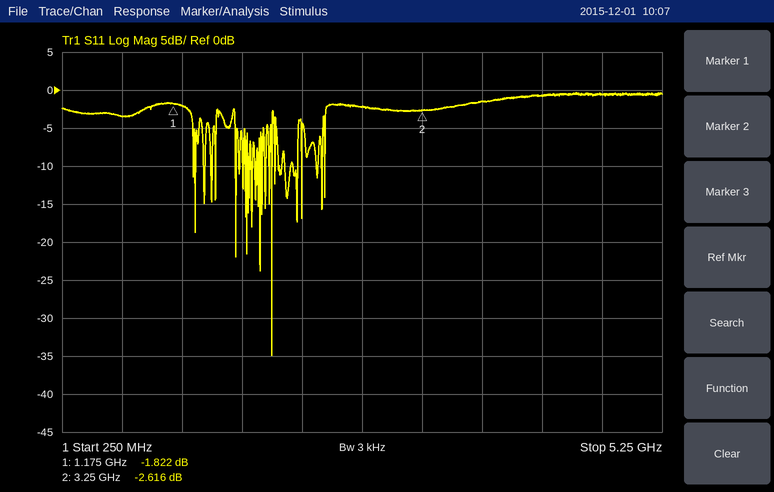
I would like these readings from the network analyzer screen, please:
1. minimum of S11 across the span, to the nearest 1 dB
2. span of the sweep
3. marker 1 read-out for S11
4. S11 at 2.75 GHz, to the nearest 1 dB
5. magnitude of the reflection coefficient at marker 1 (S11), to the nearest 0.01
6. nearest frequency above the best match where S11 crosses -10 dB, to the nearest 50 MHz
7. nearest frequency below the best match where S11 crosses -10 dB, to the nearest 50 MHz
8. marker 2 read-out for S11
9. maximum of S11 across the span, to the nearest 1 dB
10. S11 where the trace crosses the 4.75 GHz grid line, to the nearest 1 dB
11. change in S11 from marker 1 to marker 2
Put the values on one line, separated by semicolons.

-35 dB; 5 GHz; -1.822 dB; -2 dB; 0.81; 2.00 GHz; 2.00 GHz; -2.616 dB; 0 dB; -1 dB; -0.794 dB
